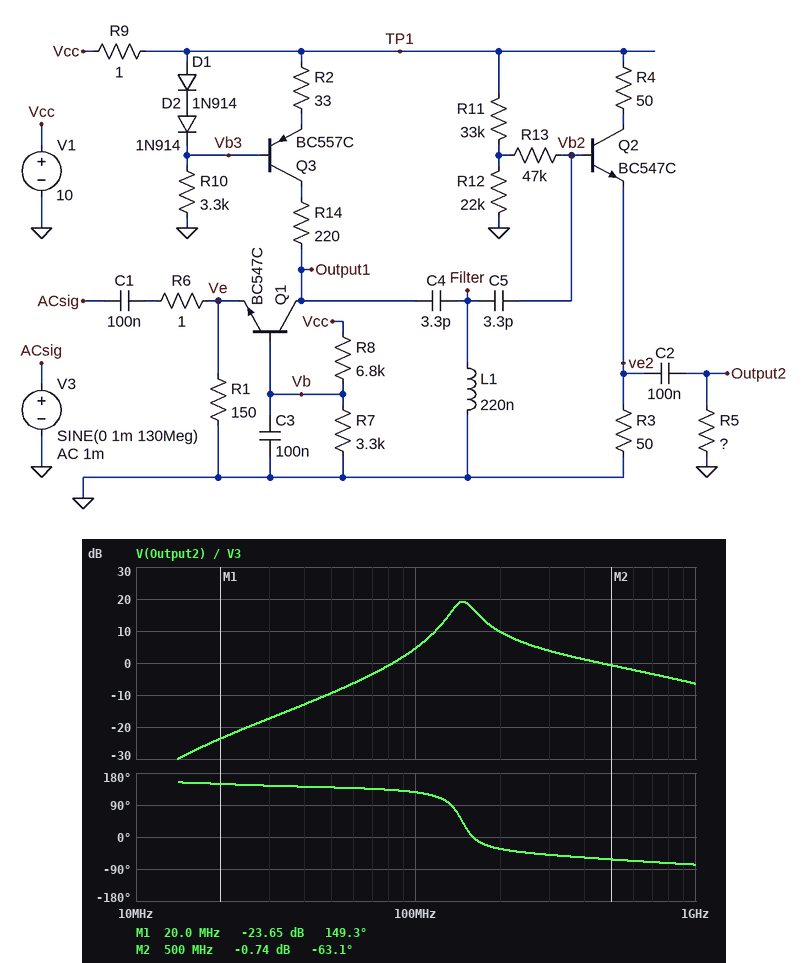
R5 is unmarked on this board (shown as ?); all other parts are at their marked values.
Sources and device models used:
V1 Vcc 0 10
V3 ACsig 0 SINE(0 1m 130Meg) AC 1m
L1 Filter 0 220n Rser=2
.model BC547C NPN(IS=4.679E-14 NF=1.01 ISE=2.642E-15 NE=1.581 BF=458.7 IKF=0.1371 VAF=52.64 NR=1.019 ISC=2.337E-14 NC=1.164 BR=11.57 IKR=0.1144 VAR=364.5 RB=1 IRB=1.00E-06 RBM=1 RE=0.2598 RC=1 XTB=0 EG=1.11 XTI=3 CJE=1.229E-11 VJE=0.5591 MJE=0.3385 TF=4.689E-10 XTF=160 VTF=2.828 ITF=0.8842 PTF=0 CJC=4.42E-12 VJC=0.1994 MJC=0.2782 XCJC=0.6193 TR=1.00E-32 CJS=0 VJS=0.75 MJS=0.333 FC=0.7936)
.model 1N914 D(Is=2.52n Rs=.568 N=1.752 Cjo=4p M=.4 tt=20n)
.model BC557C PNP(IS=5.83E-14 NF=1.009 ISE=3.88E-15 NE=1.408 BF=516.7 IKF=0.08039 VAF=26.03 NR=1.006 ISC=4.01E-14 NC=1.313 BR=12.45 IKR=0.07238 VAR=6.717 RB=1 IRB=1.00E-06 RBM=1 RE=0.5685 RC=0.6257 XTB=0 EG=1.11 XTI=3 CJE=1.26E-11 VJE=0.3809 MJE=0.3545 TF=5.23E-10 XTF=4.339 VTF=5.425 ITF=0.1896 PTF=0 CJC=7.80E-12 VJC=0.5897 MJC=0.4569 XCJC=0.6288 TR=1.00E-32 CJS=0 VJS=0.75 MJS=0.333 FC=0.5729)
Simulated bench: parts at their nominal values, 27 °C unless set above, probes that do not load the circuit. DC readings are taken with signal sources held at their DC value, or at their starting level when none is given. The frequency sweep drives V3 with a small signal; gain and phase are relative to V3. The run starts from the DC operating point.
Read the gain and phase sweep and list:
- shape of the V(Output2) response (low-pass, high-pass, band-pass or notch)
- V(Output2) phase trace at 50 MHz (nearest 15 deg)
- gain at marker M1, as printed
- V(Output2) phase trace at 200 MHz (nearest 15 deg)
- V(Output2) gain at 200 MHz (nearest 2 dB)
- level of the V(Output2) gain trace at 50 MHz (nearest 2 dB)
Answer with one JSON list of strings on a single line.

["band-pass", "135 deg", "-23.65 dB", "-30 deg", "10 dB", "-10 dB"]
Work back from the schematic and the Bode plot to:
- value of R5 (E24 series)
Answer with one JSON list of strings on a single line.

["16 Ω"]
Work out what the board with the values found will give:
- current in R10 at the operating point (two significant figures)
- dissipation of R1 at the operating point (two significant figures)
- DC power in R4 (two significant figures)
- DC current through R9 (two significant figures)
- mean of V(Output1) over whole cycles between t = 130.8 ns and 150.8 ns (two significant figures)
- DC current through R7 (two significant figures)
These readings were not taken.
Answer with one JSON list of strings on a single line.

["2.6 mA", "41 mW", "17 mW", "38 mA", "5.7 V", "960 µA"]
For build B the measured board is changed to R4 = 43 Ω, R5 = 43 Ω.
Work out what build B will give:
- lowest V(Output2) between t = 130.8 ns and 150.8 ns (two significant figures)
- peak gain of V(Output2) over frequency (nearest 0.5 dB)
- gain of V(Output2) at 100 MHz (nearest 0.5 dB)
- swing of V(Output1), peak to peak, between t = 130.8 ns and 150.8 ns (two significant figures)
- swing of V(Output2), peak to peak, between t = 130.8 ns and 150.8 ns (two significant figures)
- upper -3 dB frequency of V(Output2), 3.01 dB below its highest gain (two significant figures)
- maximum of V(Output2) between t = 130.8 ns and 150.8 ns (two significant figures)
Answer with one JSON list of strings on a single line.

["-8.8 mV", "23.5 dB", "9.5 dB", "30 mV", "18 mV", "170 MHz", "8.8 mV"]
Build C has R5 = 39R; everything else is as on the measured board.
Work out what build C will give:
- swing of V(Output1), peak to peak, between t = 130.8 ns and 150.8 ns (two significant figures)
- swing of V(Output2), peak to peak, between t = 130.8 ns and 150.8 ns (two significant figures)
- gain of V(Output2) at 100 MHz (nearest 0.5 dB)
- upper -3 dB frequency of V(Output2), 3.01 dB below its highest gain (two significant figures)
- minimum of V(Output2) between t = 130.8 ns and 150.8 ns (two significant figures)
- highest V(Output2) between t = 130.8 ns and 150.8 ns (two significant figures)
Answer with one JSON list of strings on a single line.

["29 mV", "17 mV", "9.0 dB", "170 MHz", "-8.4 mV", "8.4 mV"]
